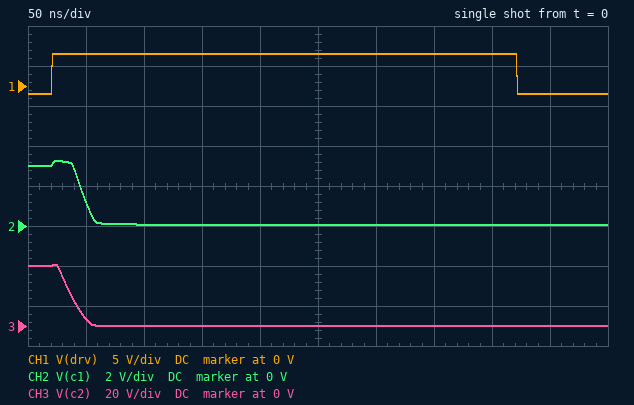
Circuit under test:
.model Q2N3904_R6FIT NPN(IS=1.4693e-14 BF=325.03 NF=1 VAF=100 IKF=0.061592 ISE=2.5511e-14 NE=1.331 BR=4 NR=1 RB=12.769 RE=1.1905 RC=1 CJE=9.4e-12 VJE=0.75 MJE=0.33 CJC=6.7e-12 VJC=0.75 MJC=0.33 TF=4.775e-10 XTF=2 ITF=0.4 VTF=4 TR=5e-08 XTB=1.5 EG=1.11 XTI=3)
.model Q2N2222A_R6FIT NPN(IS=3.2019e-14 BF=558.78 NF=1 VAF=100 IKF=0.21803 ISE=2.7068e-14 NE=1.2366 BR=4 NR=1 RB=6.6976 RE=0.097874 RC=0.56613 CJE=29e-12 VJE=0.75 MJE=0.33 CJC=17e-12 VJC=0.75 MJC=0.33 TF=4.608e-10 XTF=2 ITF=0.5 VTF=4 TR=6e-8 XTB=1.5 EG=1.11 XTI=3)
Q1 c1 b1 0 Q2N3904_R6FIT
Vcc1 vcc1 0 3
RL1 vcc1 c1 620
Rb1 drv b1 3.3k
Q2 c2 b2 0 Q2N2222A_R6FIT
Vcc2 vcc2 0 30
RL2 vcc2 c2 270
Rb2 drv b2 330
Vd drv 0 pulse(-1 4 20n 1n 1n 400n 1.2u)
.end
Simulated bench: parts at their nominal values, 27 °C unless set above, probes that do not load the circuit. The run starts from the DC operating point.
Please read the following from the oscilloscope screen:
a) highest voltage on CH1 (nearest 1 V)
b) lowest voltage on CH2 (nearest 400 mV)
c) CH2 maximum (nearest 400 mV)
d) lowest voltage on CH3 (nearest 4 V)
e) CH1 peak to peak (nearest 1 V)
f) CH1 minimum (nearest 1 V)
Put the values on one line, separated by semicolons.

4 V; 0 V; 3.2 V; 0 V; 5 V; -1 V
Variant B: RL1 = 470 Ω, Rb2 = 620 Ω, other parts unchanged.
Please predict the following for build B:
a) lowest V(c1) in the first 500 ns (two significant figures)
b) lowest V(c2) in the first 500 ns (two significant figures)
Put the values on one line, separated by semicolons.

43 mV; 140 mV
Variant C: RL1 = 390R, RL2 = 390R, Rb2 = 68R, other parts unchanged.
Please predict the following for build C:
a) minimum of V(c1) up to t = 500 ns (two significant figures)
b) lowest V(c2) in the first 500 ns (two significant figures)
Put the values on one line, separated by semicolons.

50 mV; 62 mV
